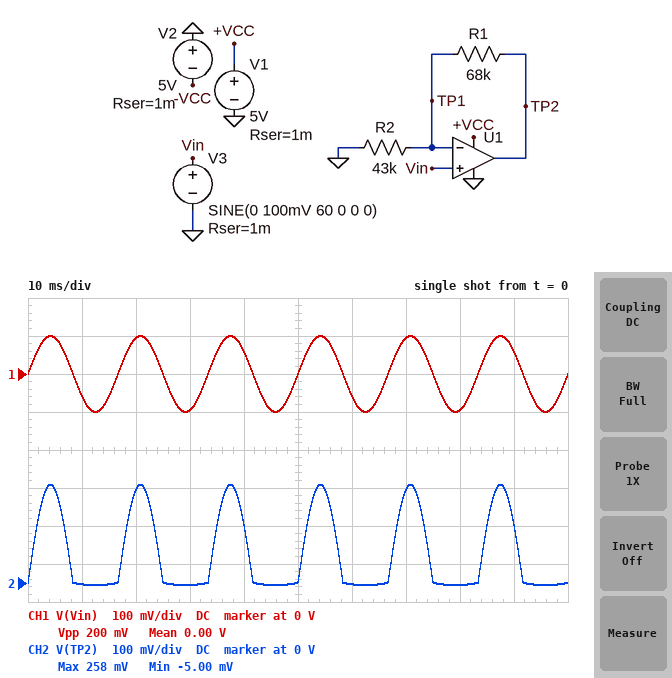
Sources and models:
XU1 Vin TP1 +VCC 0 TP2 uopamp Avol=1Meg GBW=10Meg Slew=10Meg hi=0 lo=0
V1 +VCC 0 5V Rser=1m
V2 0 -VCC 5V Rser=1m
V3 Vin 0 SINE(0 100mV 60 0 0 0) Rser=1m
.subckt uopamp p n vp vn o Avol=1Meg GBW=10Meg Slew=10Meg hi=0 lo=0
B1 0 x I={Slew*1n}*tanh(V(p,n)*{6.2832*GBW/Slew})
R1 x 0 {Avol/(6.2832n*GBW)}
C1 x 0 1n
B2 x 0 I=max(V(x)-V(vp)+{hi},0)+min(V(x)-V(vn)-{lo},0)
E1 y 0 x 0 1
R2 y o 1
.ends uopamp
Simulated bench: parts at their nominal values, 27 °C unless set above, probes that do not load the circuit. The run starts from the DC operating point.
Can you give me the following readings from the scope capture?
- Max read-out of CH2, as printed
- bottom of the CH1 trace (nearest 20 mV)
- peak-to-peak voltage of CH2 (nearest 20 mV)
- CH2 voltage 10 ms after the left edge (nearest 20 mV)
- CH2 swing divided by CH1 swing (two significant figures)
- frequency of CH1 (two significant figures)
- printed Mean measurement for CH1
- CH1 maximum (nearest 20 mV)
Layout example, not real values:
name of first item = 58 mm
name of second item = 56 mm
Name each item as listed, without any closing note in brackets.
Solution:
Max read-out of CH2, as printed = 258 mV
bottom of the CH1 trace = -100 mV
peak-to-peak voltage of CH2 = 260 mV
CH2 voltage 10 ms after the left edge = 0 V
CH2 swing divided by CH1 swing = 1.3
frequency of CH1 = 60 Hz
printed Mean measurement for CH1 = 0.00 V
CH1 maximum = 100 mV
